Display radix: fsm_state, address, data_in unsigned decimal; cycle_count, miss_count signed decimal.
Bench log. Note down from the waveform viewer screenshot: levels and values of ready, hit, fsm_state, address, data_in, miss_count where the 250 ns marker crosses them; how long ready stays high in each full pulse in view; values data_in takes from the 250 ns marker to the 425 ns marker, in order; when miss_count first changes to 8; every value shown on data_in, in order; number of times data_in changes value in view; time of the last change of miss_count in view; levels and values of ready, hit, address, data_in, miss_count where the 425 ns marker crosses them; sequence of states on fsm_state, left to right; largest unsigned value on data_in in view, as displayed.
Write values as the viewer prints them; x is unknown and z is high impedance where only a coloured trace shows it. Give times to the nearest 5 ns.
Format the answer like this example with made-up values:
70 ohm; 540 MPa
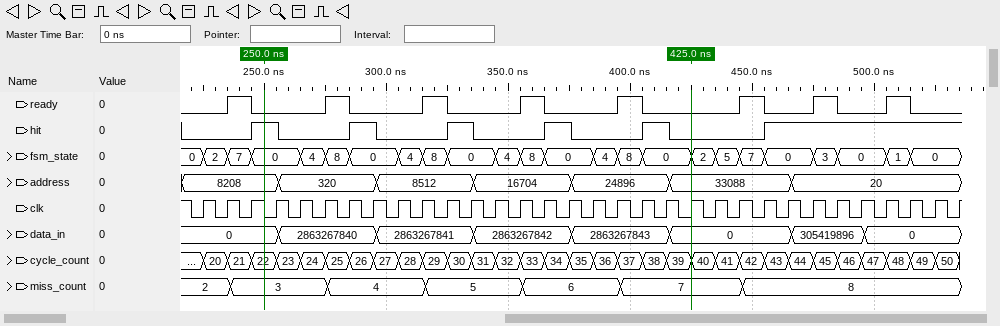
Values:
ready=0, hit=1, fsm_state=0, address=8208, data_in=0, miss_count=3; 10 ns, 10 ns, 10 ns, 10 ns, 10 ns, 10 ns, 10 ns, 10 ns; 0, 2863267840, 2863267841, 2863267842, 2863267843, 0; 445 ns; 0, 2863267840, 2863267841, 2863267842, 2863267843, 0, 305419896, 0; 7; 445 ns; ready=0, hit=0, address=33088, data_in=0, miss_count=7; 0, 2, 7, 0, 4, 8, 0, 4, 8, 0, 4, 8, 0, 4, 8, 0, 2, 5, 7, 0, 3, 0, 1, 0; 2863267843
